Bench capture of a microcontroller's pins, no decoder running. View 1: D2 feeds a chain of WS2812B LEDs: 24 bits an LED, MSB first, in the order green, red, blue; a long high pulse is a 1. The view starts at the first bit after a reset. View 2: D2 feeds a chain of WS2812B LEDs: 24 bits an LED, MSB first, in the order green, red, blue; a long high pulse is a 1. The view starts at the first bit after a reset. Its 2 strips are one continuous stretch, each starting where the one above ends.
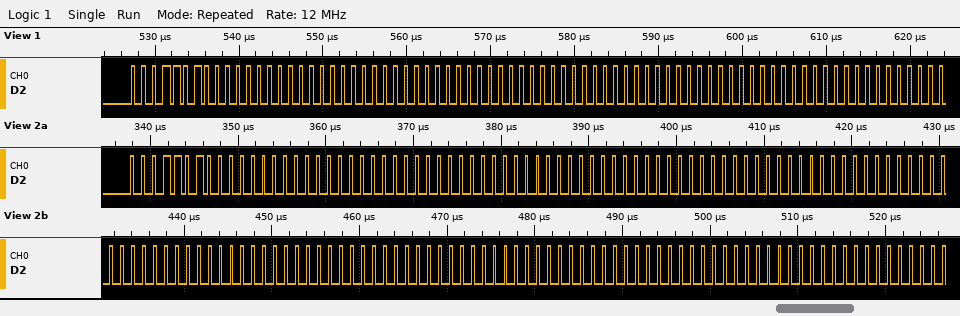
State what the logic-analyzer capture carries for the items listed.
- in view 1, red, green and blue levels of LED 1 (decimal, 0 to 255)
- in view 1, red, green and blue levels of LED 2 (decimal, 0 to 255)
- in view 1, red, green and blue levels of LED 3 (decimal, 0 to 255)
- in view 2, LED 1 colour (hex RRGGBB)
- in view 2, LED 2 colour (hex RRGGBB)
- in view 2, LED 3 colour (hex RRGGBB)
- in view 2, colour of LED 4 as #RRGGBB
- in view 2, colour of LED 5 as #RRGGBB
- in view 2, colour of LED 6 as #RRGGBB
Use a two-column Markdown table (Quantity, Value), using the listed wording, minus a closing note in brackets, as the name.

| Quantity | Value |
|---|---|
| in view 1, red, green and blue levels of LED 1 | 0, 26, 0 |
| in view 1, red, green and blue levels of LED 2 | 0, 0, 0 |
| in view 1, red, green and blue levels of LED 3 | 0, 0, 0 |
| in view 2, LED 1 colour | #001A00 |
| in view 2, LED 2 colour | #000000 |
| in view 2, LED 3 colour | #000000 |
| in view 2, colour of LED 4 as #RRGGBB | #000000 |
| in view 2, colour of LED 5 as #RRGGBB | #000000 |
| in view 2, colour of LED 6 as #RRGGBB | #000000 |
